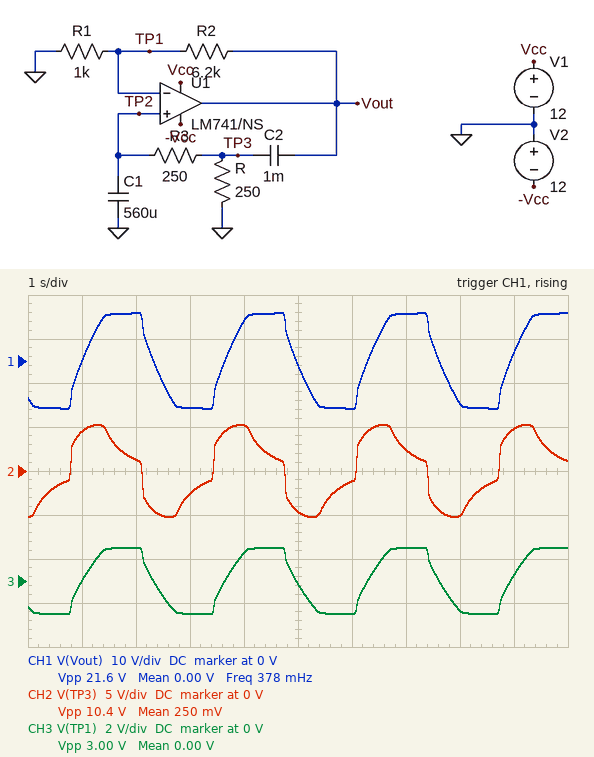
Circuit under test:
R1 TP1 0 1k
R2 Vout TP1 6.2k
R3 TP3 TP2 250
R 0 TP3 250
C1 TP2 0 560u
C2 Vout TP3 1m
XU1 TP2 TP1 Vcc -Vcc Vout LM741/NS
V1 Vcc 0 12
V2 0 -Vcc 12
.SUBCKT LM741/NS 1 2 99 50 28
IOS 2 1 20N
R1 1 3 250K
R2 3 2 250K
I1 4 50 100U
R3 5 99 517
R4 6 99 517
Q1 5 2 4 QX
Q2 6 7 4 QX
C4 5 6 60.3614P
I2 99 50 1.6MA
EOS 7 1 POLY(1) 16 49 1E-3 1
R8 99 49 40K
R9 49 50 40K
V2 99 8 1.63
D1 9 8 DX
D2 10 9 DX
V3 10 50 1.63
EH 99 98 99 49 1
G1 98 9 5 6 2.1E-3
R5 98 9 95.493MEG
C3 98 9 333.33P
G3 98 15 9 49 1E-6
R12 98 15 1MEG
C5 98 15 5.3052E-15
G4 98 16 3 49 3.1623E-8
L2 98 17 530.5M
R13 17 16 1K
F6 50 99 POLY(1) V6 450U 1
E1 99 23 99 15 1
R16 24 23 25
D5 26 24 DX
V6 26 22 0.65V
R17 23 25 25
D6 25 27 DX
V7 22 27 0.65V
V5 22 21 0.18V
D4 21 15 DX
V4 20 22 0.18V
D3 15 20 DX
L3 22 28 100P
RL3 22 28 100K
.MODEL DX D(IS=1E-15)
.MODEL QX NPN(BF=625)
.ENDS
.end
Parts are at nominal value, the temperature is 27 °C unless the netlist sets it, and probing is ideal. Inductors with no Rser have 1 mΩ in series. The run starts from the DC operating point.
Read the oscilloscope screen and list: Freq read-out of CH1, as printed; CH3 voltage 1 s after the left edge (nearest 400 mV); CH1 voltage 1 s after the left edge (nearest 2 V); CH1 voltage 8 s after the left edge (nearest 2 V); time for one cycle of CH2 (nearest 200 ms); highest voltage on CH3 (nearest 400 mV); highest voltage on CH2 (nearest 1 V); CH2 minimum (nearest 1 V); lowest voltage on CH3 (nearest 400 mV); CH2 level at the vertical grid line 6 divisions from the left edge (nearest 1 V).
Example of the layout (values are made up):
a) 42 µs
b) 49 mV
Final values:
a) 378 mHz
b) 0 V
c) 0 V
d) -10 V
e) 2.6 s
f) 1.6 V
g) 5 V
h) -5 V
i) -1.6 V
j) -1 V
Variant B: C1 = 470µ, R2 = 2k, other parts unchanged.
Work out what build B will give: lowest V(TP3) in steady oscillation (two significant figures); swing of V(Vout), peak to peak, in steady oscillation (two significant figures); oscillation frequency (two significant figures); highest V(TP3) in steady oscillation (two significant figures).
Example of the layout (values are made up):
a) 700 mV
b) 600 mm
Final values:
a) -4.9 V
b) 21 V
c) 580 mHz
d) 4.9 V
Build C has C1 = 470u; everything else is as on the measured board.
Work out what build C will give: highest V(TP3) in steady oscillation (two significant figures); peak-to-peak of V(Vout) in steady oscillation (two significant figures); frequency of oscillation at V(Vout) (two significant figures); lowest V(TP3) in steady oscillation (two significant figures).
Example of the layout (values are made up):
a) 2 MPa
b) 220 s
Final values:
a) 5.4 V
b) 22 V
c) 390 mHz
d) -5.4 V
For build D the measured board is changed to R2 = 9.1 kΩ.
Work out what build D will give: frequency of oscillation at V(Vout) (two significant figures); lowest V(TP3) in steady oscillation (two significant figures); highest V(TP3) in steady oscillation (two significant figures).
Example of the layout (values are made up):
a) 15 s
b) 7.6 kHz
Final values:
a) 340 mHz
b) -5.3 V
c) 5.3 V
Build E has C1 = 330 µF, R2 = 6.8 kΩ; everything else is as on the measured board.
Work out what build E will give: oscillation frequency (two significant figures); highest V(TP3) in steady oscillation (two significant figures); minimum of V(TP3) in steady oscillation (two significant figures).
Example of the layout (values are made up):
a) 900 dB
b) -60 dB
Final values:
a) 410 mHz
b) 5.7 V
c) -5.7 V
